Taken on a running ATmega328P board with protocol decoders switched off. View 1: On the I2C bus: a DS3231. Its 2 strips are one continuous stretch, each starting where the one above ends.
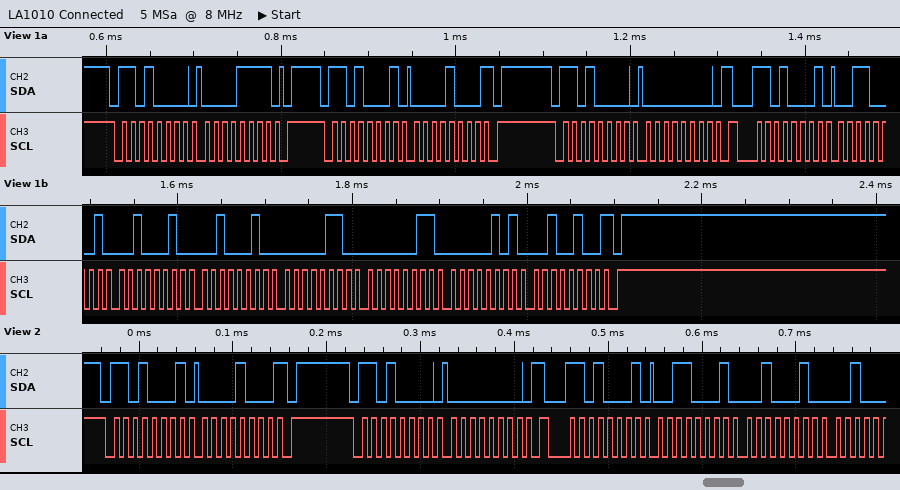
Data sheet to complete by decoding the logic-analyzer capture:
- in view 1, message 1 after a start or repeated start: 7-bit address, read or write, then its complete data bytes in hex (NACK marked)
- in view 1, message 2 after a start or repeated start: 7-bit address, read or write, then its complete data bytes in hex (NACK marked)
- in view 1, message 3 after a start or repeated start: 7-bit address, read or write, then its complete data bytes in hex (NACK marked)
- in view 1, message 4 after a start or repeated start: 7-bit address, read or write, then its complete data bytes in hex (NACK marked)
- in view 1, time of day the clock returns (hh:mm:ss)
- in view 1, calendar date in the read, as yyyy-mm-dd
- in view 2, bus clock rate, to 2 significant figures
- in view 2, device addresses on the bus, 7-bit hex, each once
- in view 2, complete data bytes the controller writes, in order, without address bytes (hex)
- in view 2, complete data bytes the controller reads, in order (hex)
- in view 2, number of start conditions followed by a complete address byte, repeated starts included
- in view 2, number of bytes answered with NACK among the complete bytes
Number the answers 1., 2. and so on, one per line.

1. 0x68 write: 0F
2. 0x68 read: 08 NACK
3. 0x68 write: 00
4. 0x68 read: 31 22 22 06 03 05 24 NACK
5. 22:22:31
6. 2024-05-03
7. 100 kHz
8. 0x68
9. 00
10. 08 31 22
11. 3
12. 1
